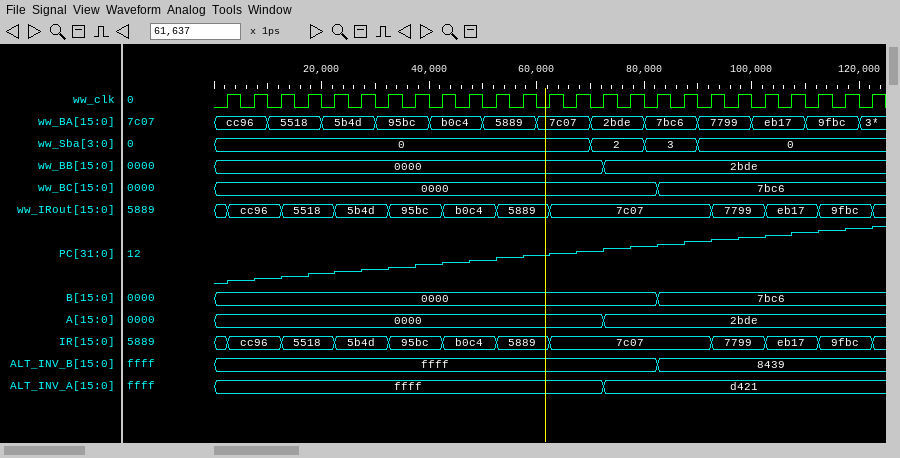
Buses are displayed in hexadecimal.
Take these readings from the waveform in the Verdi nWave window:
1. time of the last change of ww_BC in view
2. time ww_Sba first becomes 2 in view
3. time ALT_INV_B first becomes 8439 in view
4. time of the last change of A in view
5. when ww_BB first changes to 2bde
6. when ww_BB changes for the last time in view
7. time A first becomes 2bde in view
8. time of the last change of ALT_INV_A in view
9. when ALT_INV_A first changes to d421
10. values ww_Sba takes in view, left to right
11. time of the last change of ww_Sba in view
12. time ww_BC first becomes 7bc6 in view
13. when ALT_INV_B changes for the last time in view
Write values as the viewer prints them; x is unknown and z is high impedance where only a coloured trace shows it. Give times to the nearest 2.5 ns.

82.5 ns
70 ns
82.5 ns
72.5 ns
72.5 ns
72.5 ns
72.5 ns
72.5 ns
72.5 ns
0, 2, 3, 0
90 ns
82.5 ns
82.5 ns
